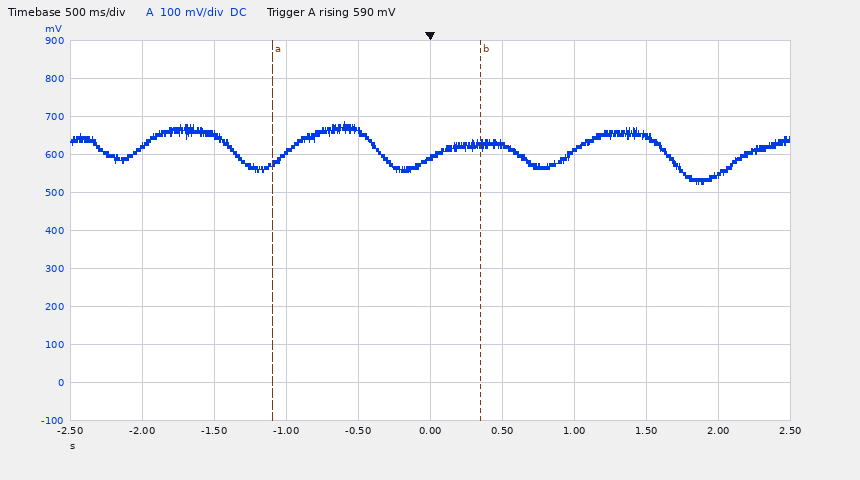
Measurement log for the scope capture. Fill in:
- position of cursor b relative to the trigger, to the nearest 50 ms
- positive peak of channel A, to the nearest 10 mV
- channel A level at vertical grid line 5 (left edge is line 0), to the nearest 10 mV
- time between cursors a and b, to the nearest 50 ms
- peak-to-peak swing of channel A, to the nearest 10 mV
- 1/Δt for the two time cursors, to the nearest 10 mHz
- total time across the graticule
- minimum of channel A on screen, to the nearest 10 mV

+350 ms
690 mV
590 mV
1.45 s
170 mV
690 mHz
5 s
520 mV
